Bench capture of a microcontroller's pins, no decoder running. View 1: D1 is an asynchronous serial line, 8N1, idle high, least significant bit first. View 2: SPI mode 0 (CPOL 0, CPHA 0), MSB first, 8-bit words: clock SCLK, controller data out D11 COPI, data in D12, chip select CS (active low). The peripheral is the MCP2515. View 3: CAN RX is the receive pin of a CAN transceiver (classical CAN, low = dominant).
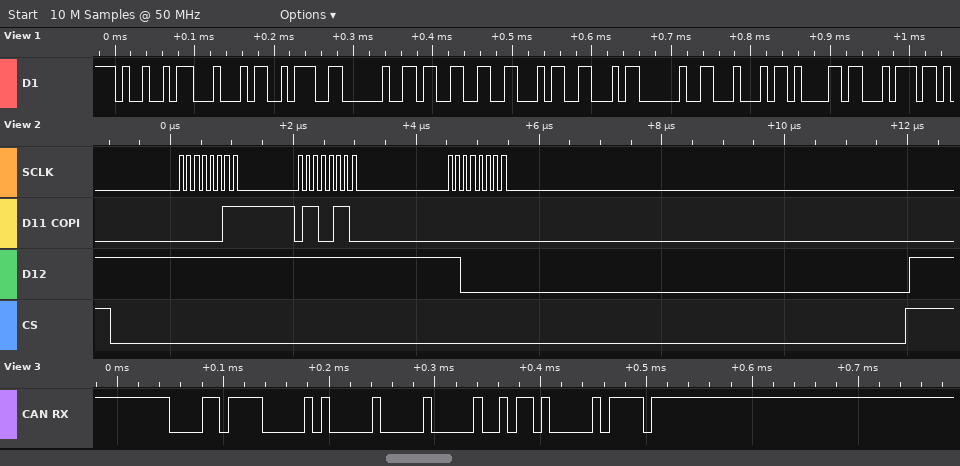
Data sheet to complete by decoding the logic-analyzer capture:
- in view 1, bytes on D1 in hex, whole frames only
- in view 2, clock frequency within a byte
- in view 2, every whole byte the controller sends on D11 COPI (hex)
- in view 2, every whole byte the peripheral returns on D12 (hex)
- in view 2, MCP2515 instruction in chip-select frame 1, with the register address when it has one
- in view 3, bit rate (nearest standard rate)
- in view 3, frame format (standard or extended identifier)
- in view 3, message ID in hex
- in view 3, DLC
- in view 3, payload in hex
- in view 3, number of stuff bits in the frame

49 44 3A 20 33 46 46 20 44 61 74
8 MHz
03 66 00
FF FF C0
READ 0x66
125 kbit/s
standard
0x0DE
2
00 00
5
